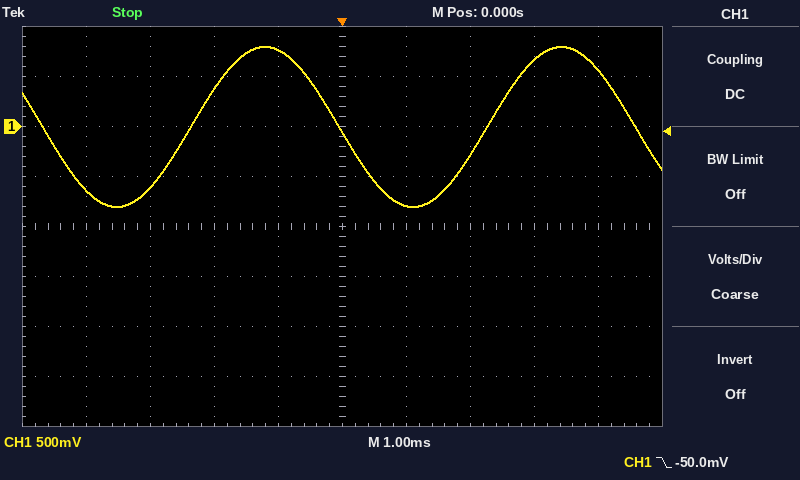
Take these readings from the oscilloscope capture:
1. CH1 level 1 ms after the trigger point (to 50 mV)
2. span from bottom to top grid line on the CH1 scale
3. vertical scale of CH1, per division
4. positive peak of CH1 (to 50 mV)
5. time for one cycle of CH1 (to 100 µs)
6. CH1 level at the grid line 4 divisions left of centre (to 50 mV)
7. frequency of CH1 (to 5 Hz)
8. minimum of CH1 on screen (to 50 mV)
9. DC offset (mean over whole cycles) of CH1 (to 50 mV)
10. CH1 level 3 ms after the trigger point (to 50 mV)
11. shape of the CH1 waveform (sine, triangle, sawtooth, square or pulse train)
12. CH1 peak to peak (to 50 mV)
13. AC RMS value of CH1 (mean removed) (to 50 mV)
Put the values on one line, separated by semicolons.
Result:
-800 mV; 4 V; 500 mV; 800 mV; 4.6 ms; -650 mV; 215 Hz; -800 mV; 0 mV; 650 mV; sine; 1.60 V; 550 mV
